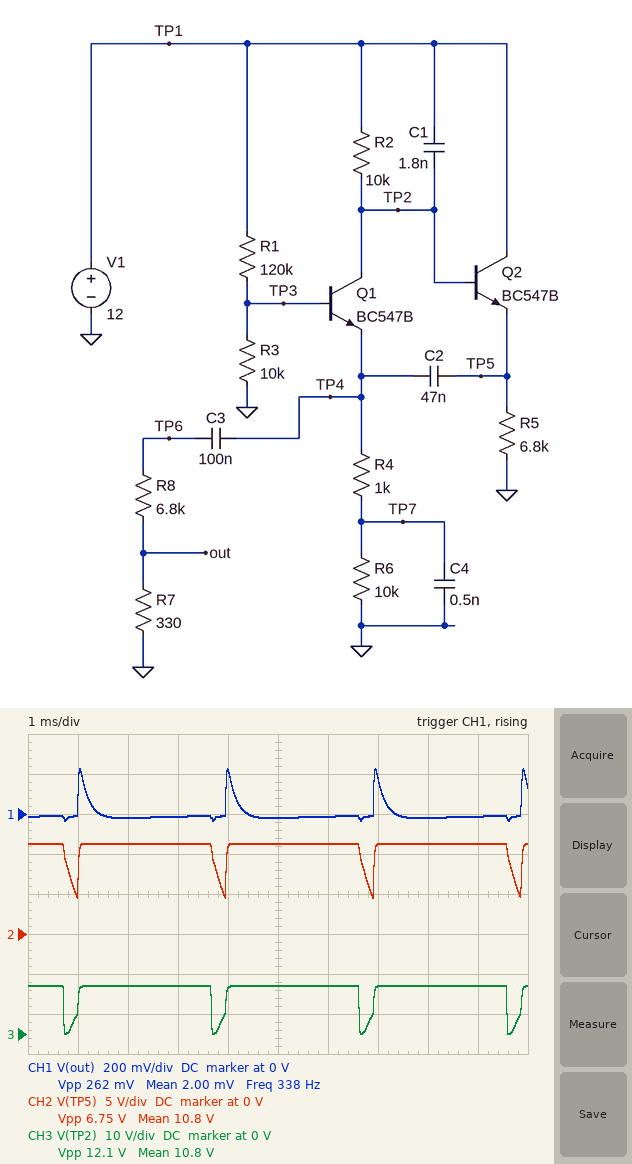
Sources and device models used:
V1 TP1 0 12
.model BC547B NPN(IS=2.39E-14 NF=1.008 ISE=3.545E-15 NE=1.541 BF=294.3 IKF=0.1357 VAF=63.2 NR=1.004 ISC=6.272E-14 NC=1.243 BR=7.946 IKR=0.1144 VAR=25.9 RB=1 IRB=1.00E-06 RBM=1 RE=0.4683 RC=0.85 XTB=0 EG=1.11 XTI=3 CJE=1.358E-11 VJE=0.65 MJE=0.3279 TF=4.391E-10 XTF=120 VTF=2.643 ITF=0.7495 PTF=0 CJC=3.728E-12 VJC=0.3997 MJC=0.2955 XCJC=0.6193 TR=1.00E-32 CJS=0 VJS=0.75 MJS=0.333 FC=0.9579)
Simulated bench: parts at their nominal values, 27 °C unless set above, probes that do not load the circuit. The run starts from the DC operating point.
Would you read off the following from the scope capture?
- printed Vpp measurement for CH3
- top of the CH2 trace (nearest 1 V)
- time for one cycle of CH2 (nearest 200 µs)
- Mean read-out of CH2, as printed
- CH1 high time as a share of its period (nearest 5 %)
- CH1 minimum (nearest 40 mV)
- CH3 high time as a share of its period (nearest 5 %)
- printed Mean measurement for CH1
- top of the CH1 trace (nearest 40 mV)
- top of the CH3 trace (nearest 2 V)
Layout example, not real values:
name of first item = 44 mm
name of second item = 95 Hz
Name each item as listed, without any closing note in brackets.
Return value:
printed Vpp measurement for CH3 = 12.1 V
top of the CH2 trace = 11 V
time for one cycle of CH2 = 3.0 ms
Mean read-out of CH2, as printed = 10.8 V
CH1 high time as a share of its period = 5 %
CH1 minimum = -40 mV
CH3 high time as a share of its period = 90 %
printed Mean measurement for CH1 = 2.00 mV
top of the CH1 trace = 240 mV
top of the CH3 trace = 12 V
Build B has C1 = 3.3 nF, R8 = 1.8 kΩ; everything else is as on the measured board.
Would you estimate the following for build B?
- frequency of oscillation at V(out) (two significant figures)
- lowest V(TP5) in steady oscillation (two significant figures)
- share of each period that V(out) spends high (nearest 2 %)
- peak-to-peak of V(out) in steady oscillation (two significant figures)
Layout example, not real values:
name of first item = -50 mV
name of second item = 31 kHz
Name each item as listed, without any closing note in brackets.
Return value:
frequency of oscillation at V(out) = 320 Hz
lowest V(TP5) in steady oscillation = 4.3 V
share of each period that V(out) spends high = 4 %
peak-to-peak of V(out) in steady oscillation = 550 mV
